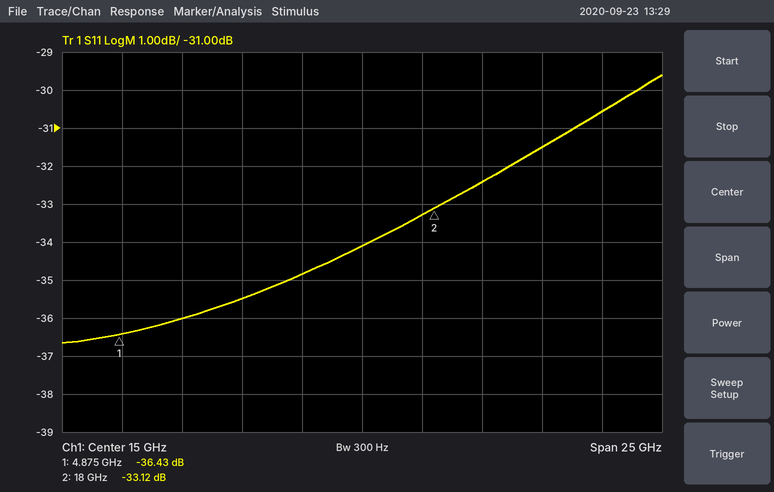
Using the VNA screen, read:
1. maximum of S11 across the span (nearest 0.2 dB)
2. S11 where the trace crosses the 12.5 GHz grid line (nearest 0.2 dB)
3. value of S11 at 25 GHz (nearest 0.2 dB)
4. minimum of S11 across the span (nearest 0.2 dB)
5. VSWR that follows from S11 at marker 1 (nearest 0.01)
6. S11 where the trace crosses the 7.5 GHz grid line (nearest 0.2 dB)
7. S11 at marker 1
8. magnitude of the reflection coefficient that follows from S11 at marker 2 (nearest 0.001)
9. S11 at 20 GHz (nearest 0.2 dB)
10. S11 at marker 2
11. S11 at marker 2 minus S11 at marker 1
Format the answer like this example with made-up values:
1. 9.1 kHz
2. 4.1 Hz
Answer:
1. -29.6 dB
2. -34.8 dB
3. -30.6 dB
4. -36.6 dB
5. 1.03
6. -36.0 dB
7. -36.43 dB
8. 0.022
9. -32.4 dB
10. -33.12 dB
11. 3.31 dB
